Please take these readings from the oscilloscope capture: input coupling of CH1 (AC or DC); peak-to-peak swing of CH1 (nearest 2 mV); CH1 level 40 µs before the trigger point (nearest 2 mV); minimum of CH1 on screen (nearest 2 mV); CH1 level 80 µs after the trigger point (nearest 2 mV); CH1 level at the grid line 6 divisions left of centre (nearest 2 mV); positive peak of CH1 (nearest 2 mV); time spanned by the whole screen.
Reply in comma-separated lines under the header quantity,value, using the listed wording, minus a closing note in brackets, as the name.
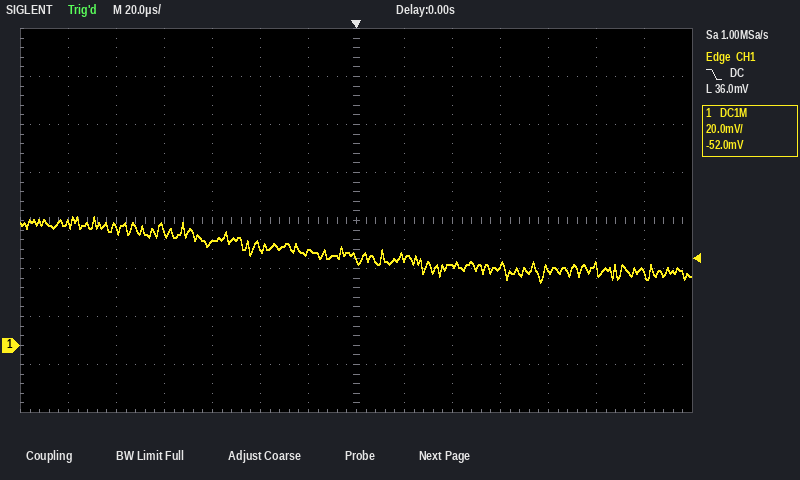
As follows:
quantity,value
input coupling of CH1,DC
peak-to-peak swing of CH1,28 mV
CH1 level 40 µs before the trigger point,40 mV
minimum of CH1 on screen,26 mV
CH1 level 80 µs after the trigger point,32 mV
CH1 level at the grid line 6 divisions left of centre,50 mV
positive peak of CH1,54 mV
time spanned by the whole screen,280 µs
